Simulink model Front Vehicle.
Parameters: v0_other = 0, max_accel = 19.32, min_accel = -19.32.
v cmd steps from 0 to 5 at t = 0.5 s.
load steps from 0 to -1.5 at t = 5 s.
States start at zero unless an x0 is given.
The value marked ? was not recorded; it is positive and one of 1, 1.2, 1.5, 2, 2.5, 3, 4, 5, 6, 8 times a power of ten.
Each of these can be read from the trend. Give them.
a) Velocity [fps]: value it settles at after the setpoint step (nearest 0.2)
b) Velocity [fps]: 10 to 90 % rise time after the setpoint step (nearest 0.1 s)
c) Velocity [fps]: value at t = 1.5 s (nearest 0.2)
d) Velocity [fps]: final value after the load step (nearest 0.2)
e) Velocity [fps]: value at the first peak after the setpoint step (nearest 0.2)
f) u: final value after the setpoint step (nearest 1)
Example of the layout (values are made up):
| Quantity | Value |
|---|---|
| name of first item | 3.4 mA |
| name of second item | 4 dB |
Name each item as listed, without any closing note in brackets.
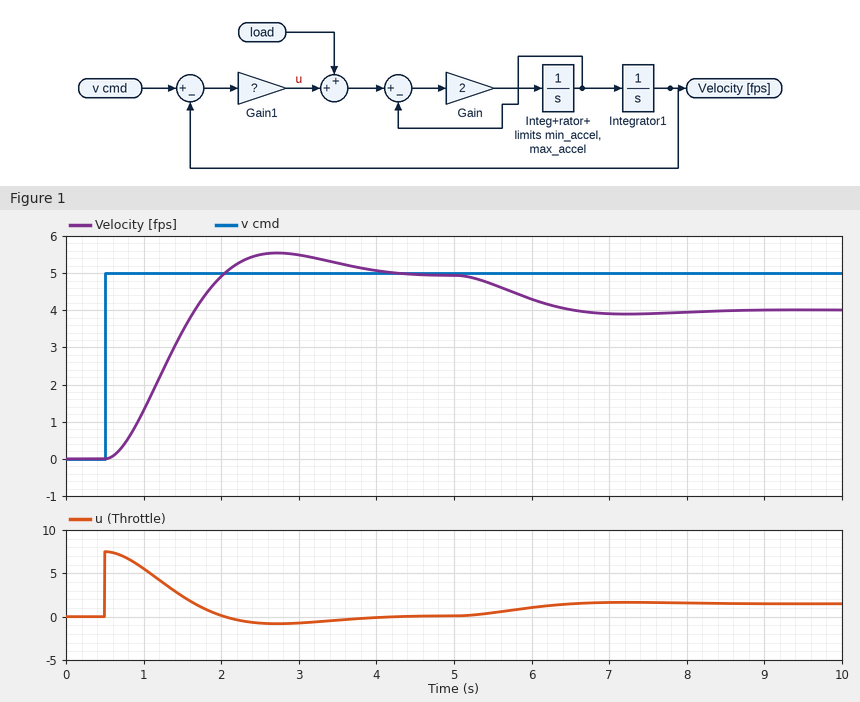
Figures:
| Quantity | Value |
|---|---|
| Velocity [fps]: value it settles at after the setpoint step | 5.0 |
| Velocity [fps]: 10 to 90 % rise time after the setpoint step | 1.0 s |
| Velocity [fps]: value at t = 1.5 s | 3.4 |
| Velocity [fps]: final value after the load step | 4.0 |
| Velocity [fps]: value at the first peak after the setpoint step | 5.6 |
| u: final value after the setpoint step | 0 |
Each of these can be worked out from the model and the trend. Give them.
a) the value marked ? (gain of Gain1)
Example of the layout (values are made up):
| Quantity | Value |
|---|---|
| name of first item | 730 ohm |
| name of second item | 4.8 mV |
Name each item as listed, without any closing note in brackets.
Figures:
| Quantity | Value |
|---|---|
| the value marked ? | 1.5 |
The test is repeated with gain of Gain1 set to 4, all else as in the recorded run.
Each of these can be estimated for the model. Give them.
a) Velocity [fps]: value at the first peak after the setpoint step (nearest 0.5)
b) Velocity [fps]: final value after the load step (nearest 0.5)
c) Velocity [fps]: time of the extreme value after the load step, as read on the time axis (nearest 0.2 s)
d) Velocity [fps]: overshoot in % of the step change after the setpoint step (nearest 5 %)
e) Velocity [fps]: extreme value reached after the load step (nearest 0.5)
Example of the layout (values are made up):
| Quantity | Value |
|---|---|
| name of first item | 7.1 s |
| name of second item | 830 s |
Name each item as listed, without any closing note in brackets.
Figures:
| Quantity | Value |
|---|---|
| Velocity [fps]: value at the first peak after the setpoint step | 6.5 |
| Velocity [fps]: final value after the load step | 4.5 |
| Velocity [fps]: time of the extreme value after the load step, as read on the time axis | 6.2 s |
| Velocity [fps]: overshoot in % of the step change after the setpoint step | 30 % |
| Velocity [fps]: extreme value reached after the load step | 4.5 |
